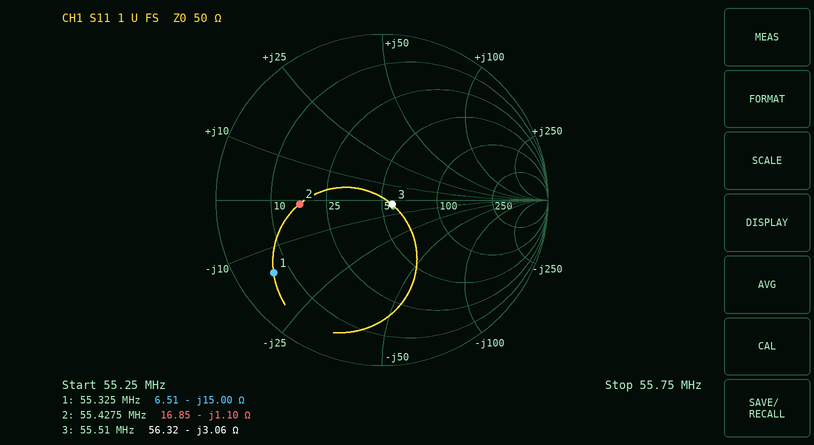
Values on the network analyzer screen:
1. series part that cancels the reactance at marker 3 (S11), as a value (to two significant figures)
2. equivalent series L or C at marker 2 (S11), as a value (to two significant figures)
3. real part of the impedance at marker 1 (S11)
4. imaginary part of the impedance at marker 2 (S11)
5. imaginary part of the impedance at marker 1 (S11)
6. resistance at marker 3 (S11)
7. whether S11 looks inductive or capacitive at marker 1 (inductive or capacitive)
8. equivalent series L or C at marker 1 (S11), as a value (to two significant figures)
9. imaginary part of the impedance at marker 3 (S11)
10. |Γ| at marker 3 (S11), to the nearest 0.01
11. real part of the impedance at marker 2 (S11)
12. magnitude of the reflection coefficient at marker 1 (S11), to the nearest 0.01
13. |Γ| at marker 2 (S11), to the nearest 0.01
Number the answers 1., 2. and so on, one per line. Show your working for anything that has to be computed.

1. L = 3.06 Ω/(2π × 55.51 MHz) ≈ 8.8 nH
2. C = 1/(2π × 55.4275 MHz × 1.1 Ω) ≈ 2.6 nF
3. 6.51 Ω
4. -1.10 Ω
5. -15.00 Ω
6. 56.32 Ω
7. capacitive
8. C = 1/(2π × 55.325 MHz × 15 Ω) ≈ 192 pF, so 190 pF to two significant figures
9. -3.06 Ω
10. 0.07
11. 16.85 Ω
12. 0.79
13. 0.50
